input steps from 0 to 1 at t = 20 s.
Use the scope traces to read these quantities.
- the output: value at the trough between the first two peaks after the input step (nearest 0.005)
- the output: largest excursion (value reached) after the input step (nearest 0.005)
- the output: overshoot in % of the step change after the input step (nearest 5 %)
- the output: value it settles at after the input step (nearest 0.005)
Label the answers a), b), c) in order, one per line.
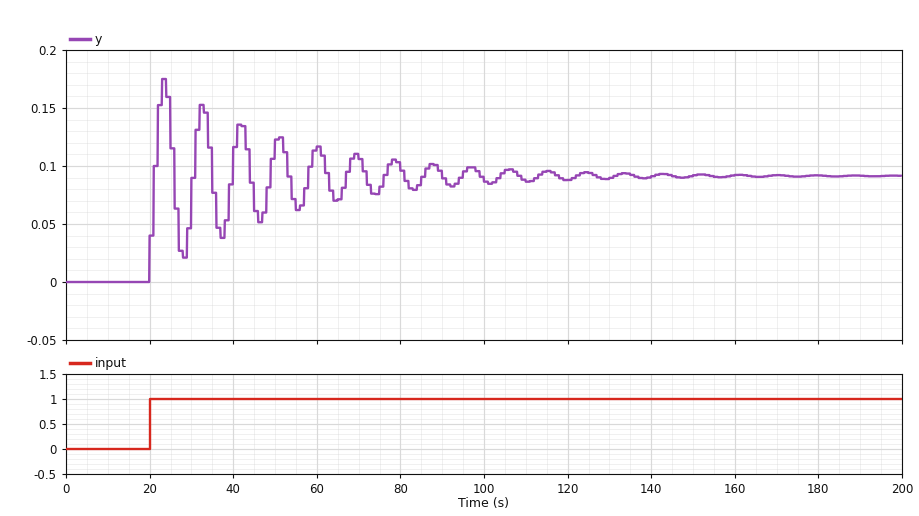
a) 0.020
b) 0.175
c) 90 %
d) 0.090
